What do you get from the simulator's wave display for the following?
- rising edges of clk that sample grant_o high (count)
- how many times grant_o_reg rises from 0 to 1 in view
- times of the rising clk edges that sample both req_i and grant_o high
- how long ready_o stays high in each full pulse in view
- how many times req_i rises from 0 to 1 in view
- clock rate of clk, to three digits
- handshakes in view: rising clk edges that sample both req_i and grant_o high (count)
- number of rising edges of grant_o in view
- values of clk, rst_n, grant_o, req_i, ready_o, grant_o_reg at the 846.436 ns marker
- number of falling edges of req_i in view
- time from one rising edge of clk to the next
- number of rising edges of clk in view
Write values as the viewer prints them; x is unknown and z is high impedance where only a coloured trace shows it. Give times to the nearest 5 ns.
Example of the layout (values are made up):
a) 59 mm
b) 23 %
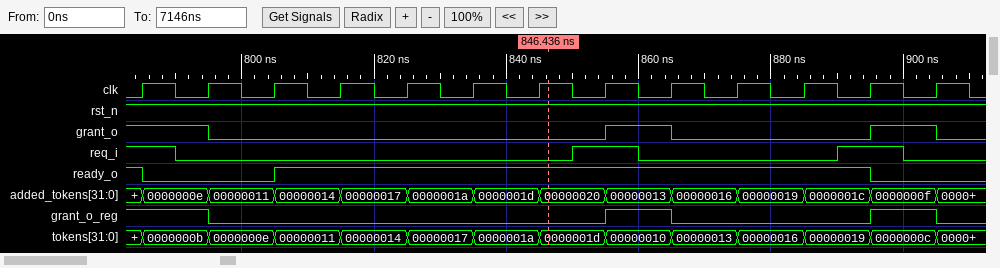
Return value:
a) 4
b) 2
c) 785 ns
d) 90 ns
e) 2
f) 100 MHz
g) 1
h) 2
i) clk=1, rst_n=1, grant_o=0, req_i=0, ready_o=1, grant_o_reg=0
j) 3
k) 10 ns
l) 13
